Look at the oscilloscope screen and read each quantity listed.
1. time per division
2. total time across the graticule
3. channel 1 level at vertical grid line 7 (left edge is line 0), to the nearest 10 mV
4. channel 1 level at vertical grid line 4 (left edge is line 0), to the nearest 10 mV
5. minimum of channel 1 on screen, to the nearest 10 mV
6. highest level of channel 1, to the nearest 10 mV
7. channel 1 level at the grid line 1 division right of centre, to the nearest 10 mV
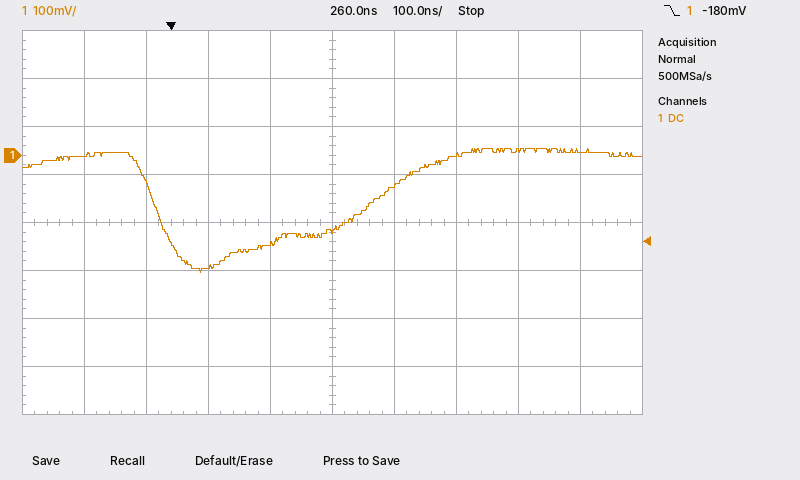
100 ns
1 µs
0 mV
-180 mV
-240 mV
10 mV
-60 mV
